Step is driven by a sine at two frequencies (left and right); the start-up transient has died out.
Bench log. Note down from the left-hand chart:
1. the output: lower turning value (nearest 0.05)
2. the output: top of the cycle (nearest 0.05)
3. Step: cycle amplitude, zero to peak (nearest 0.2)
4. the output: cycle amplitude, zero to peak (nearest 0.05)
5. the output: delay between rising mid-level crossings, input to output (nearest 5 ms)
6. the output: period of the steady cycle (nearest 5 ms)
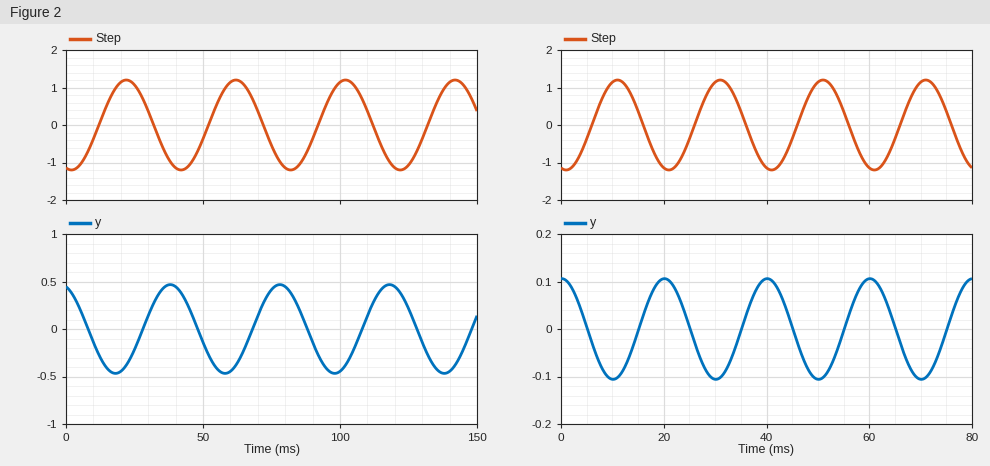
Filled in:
-0.45
0.45
1.2
0.45
15 ms
40 ms
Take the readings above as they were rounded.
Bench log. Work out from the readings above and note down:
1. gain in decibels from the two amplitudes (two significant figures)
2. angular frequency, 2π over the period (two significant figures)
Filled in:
-8.5 dB
0.16 rad/ms
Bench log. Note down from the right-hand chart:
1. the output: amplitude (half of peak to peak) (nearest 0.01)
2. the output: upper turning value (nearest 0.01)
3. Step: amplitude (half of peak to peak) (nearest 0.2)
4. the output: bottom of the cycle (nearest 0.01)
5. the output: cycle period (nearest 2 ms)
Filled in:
0.11
0.11
1.2
-0.11
20 ms
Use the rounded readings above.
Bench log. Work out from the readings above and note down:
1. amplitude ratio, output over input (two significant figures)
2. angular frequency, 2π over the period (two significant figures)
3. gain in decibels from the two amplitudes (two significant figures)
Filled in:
0.092
0.31 rad/ms
-21 dB
